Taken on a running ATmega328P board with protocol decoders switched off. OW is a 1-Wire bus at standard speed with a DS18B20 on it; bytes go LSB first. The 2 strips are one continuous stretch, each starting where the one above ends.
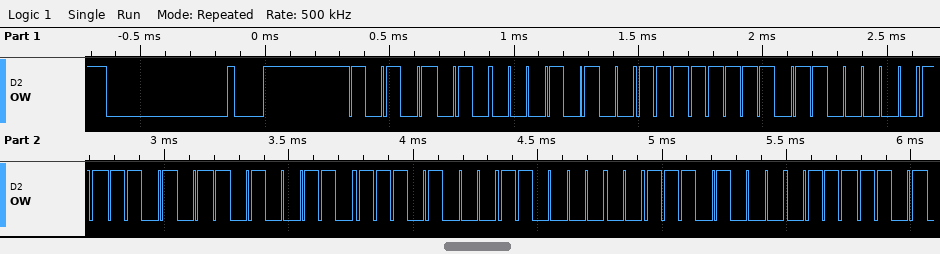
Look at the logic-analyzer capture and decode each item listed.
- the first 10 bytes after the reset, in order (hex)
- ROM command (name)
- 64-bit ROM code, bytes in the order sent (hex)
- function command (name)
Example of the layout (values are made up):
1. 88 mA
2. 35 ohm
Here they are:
1. 55 28 FF 06 AF 65 17 03 17 BE
2. Match ROM
3. 28 FF 06 AF 65 17 03 17
4. Read Scratchpad
